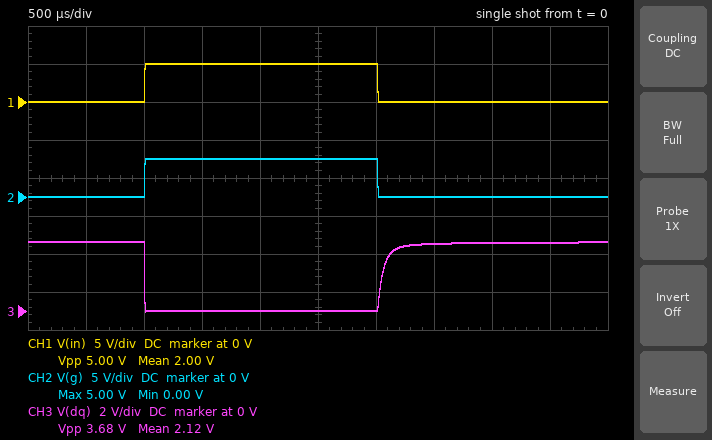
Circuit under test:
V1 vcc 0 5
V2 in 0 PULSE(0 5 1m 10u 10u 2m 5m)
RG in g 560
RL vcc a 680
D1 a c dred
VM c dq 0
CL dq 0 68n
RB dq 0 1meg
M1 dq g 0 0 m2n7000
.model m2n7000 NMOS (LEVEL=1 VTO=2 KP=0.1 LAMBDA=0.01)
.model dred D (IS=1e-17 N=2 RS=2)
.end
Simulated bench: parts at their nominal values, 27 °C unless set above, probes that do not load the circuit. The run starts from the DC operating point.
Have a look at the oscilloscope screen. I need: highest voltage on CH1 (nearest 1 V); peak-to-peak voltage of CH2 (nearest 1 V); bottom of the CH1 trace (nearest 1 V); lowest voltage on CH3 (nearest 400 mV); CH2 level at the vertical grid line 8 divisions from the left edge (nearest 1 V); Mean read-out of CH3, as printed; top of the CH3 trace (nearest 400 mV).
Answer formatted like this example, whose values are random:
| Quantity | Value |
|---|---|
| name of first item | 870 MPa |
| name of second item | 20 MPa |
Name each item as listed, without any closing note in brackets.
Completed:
| Quantity | Value |
|---|---|
| highest voltage on CH1 | 5 V |
| peak-to-peak voltage of CH2 | 5 V |
| bottom of the CH1 trace | 0 V |
| lowest voltage on CH3 | 0 V |
| CH2 level at the vertical grid line 8 divisions from the left edge | 0 V |
| Mean read-out of CH3, as printed | 2.12 V |
| top of the CH3 trace | 3.6 V |
